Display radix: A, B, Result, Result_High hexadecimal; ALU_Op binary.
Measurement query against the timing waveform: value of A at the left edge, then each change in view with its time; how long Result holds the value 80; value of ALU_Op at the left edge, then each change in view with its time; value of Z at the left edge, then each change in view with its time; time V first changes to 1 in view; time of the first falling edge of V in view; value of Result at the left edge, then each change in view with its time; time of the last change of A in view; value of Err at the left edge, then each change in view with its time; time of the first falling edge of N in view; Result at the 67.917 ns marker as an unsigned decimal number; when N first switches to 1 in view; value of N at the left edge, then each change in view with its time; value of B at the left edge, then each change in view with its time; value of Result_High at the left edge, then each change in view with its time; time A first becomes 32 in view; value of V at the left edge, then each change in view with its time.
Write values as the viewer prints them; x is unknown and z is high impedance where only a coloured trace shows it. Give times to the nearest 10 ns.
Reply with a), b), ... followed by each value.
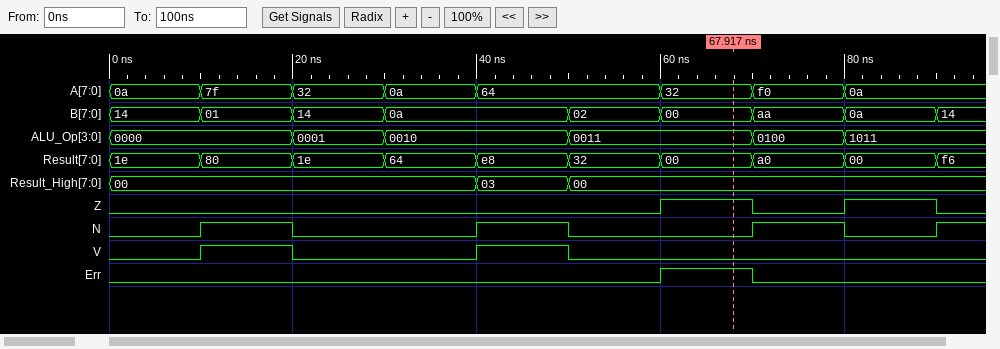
a) 0a, 7f at 10 ns, 32 at 20 ns, 0a at 30 ns, 64 at 40 ns, 32 at 60 ns, f0 at 70 ns, 0a at 80 ns
b) 10 ns
c) 0000, 0001 at 20 ns, 0010 at 30 ns, 0011 at 50 ns, 0100 at 70 ns, 1011 at 80 ns
d) 0, 1 at 60 ns, 0 at 70 ns, 1 at 80 ns, 0 at 90 ns
e) 10 ns
f) 20 ns
g) 1e, 80 at 10 ns, 1e at 20 ns, 64 at 30 ns, e8 at 40 ns, 32 at 50 ns, 00 at 60 ns, a0 at 70 ns, 00 at 80 ns, f6 at 90 ns
h) 80 ns
i) 0, 1 at 60 ns, 0 at 70 ns
j) 20 ns
k) 0
l) 10 ns
m) 0, 1 at 10 ns, 0 at 20 ns, 1 at 40 ns, 0 at 50 ns, 1 at 70 ns, 0 at 80 ns, 1 at 90 ns
n) 14, 01 at 10 ns, 14 at 20 ns, 0a at 30 ns, 02 at 50 ns, 00 at 60 ns, aa at 70 ns, 0a at 80 ns, 14 at 90 ns
o) 00, 03 at 40 ns, 00 at 50 ns
p) 20 ns
q) 0, 1 at 10 ns, 0 at 20 ns, 1 at 40 ns, 0 at 50 ns
